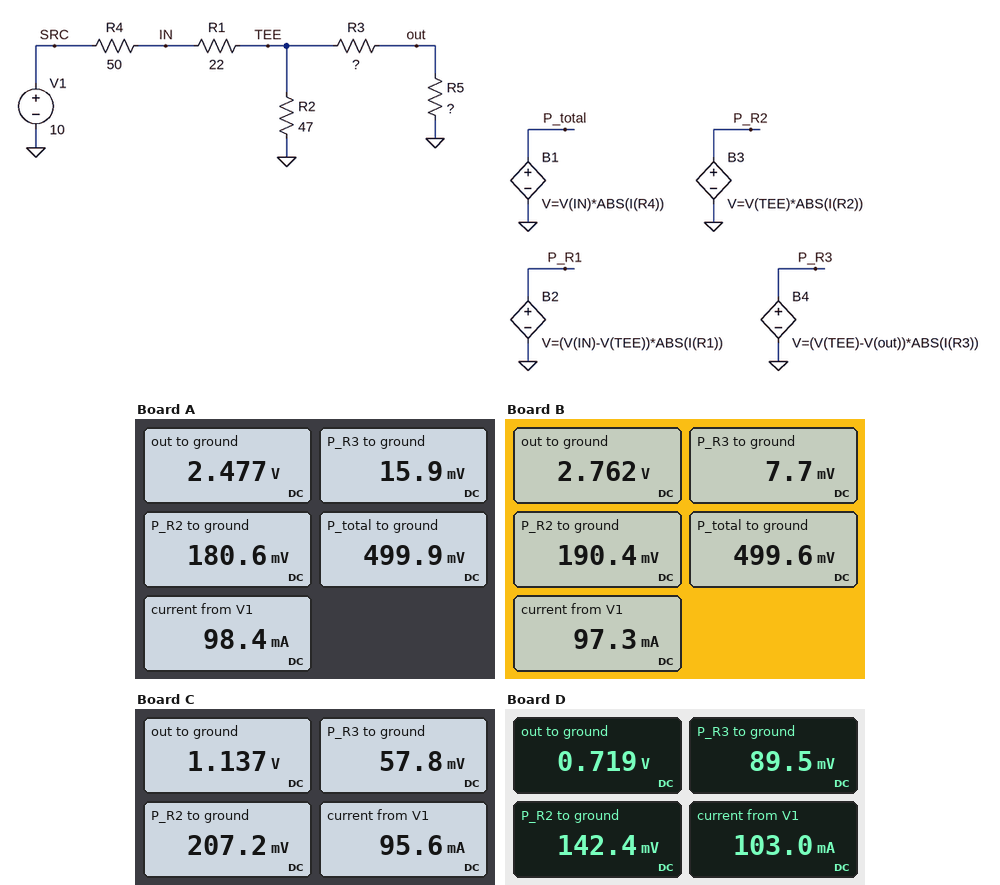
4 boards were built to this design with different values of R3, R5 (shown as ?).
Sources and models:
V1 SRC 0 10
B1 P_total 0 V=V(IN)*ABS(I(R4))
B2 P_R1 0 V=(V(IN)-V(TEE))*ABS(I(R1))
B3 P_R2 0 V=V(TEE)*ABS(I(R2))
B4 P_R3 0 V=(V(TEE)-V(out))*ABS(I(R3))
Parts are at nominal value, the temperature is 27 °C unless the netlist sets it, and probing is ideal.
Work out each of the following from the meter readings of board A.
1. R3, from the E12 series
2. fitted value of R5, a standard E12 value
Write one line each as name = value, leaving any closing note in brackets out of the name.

R3, from the E12 series = 12 Ω
fitted value of R5, a standard E12 value = 68 Ω
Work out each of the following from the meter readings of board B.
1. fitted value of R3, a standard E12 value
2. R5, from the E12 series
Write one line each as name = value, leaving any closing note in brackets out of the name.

fitted value of R3, a standard E12 value = 6.8 Ω
R5, from the E12 series = 82 Ω
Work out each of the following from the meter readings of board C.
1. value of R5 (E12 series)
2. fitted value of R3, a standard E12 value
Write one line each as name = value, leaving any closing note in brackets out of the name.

value of R5 = 39 Ω
fitted value of R3, a standard E12 value = 68 Ω
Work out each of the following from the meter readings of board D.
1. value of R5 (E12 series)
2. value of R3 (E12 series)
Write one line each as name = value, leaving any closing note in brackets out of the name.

value of R5 = 15 Ω
value of R3 = 39 Ω
